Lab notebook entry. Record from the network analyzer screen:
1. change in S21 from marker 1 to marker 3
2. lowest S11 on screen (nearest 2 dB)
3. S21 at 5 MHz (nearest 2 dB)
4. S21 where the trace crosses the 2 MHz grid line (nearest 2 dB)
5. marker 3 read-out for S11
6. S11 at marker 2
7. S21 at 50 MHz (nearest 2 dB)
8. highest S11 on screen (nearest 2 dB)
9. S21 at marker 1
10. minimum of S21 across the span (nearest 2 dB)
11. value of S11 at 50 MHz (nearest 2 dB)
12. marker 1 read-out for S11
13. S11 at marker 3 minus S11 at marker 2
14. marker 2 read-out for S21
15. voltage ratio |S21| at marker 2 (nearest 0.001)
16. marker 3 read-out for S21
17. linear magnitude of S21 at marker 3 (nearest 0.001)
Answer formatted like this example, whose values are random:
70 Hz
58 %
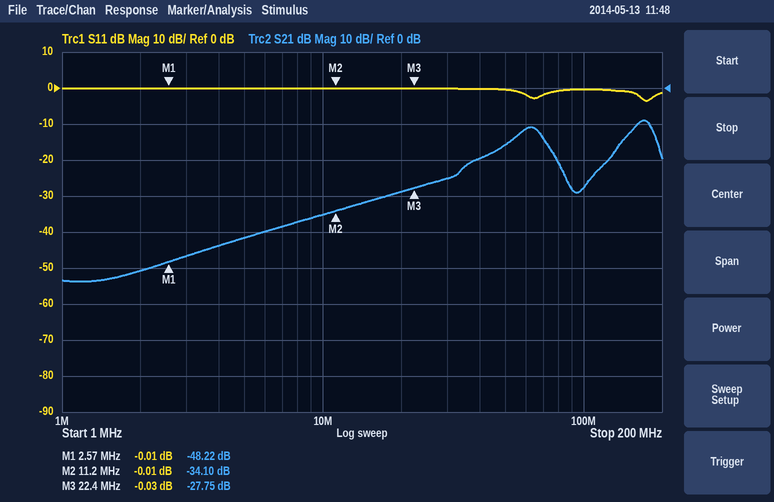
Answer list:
20.47 dB
-4 dB
-42 dB
-50 dB
-0.03 dB
-0.01 dB
-16 dB
0 dB
-48.22 dB
-54 dB
0 dB
-0.01 dB
-0.02 dB
-34.10 dB
0.020
-27.75 dB
0.041
